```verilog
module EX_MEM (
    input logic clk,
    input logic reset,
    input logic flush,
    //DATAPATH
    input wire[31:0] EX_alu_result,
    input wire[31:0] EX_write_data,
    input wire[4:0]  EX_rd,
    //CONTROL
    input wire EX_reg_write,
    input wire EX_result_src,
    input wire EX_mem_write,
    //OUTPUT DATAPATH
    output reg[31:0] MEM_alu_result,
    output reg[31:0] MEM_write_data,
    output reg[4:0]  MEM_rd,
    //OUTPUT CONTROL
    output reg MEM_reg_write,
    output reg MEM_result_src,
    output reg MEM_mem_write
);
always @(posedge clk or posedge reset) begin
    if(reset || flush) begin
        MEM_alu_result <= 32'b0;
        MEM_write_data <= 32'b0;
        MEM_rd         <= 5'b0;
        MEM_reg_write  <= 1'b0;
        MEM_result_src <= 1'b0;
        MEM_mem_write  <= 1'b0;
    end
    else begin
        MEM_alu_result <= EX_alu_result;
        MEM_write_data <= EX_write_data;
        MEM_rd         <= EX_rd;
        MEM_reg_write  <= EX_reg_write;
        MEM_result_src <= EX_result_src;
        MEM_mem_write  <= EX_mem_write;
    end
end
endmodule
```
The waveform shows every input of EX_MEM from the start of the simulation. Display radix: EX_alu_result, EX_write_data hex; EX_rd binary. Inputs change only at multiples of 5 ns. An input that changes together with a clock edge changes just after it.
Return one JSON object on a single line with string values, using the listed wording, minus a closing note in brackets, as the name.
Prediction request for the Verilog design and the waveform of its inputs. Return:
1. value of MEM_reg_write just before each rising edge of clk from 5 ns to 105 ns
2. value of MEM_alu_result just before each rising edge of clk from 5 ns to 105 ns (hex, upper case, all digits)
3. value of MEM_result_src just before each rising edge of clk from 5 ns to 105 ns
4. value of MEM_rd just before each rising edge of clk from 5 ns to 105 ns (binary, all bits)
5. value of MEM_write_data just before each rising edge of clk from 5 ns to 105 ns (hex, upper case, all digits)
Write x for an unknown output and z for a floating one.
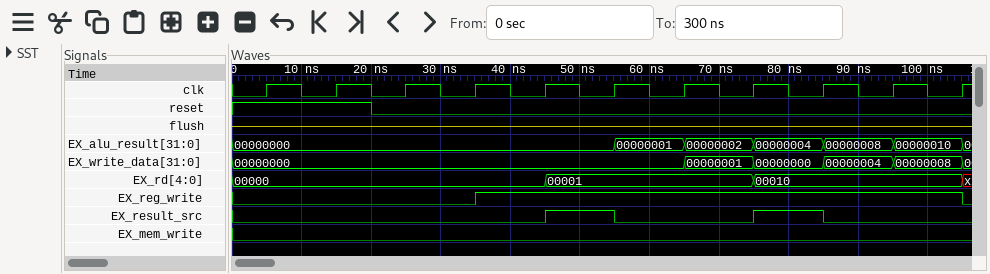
{"value of MEM_reg_write just before each rising edge of clk from 5 ns to 105 ns": "0 0 0 0 0 1 1 1 1 1 1", "value of MEM_alu_result just before each rising edge of clk from 5 ns to 105 ns": "00000000, 00000000, 00000000, 00000000, 00000000, 00000000, 00000000, 00000001, 00000002, 00000004, 00000008", "value of MEM_result_src just before each rising edge of clk from 5 ns to 105 ns": "0 0 0 0 0 0 1 0 0 1 0", "value of MEM_rd just before each rising edge of clk from 5 ns to 105 ns": "00000, 00000, 00000, 00000, 00000, 00000, 00001, 00001, 00001, 00010, 00010", "value of MEM_write_data just before each rising edge of clk from 5 ns to 105 ns": "00000000, 00000000, 00000000, 00000000, 00000000, 00000000, 00000000, 00000000, 00000001, 00000000, 00000004"}
